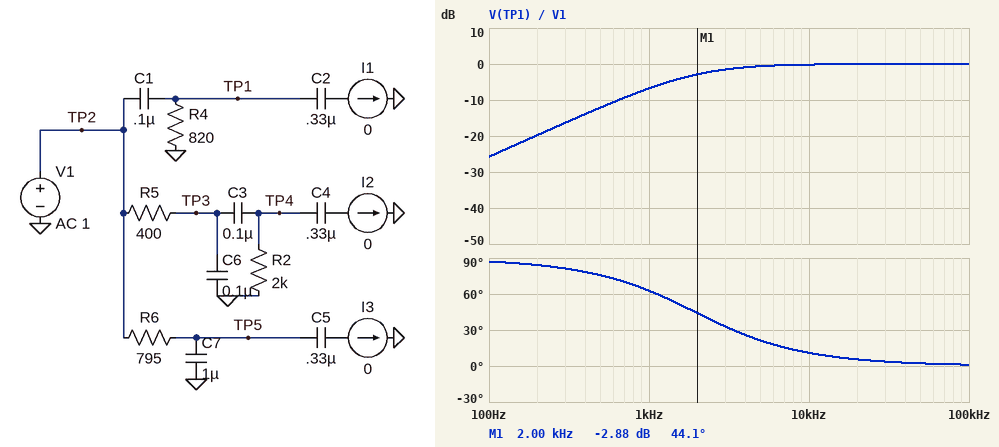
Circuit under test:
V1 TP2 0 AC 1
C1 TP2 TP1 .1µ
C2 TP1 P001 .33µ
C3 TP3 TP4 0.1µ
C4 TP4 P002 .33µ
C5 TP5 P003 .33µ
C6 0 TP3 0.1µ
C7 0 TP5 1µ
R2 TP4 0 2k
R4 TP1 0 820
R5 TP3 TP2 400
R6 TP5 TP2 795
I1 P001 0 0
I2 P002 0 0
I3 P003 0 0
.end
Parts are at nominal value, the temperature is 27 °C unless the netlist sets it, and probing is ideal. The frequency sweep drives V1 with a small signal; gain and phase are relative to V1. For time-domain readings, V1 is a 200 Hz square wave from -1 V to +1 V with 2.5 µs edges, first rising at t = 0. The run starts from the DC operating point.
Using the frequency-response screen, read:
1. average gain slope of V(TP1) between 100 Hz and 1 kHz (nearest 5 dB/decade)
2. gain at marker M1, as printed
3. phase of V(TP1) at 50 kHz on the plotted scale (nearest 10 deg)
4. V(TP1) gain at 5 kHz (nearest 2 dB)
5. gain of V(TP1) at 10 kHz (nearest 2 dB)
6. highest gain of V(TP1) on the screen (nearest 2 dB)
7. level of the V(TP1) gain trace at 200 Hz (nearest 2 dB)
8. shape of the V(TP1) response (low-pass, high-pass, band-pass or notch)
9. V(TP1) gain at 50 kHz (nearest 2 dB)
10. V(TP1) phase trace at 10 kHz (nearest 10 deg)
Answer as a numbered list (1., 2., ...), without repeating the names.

1. 20 dB/decade
2. -2.88 dB
3. 0 deg
4. 0 dB
5. 0 dB
6. 0 dB
7. -20 dB
8. high-pass
9. 0 dB
10. 10 deg
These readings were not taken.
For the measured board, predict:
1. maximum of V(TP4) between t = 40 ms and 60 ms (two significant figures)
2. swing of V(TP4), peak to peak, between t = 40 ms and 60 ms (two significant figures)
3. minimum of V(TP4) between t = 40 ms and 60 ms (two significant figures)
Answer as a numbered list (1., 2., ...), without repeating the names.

1. 1.2 V
2. 2.4 V
3. -1.2 V
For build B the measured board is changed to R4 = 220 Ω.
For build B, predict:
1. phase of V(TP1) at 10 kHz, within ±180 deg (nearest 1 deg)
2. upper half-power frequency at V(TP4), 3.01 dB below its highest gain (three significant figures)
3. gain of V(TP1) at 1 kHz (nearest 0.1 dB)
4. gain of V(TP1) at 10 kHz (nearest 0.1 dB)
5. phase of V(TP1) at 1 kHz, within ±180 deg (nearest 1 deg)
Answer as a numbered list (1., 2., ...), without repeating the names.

1. 36 deg
2. 6.09 kHz
3. -17.3 dB
4. -1.8 dB
5. 82 deg
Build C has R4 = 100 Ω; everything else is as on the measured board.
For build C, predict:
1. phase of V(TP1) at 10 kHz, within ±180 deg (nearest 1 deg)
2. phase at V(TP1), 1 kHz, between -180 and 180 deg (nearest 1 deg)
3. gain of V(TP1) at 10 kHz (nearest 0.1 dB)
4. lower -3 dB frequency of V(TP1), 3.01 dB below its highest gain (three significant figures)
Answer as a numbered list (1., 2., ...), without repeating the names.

1. 58 deg
2. 86 deg
3. -5.5 dB
4. 15.9 kHz
